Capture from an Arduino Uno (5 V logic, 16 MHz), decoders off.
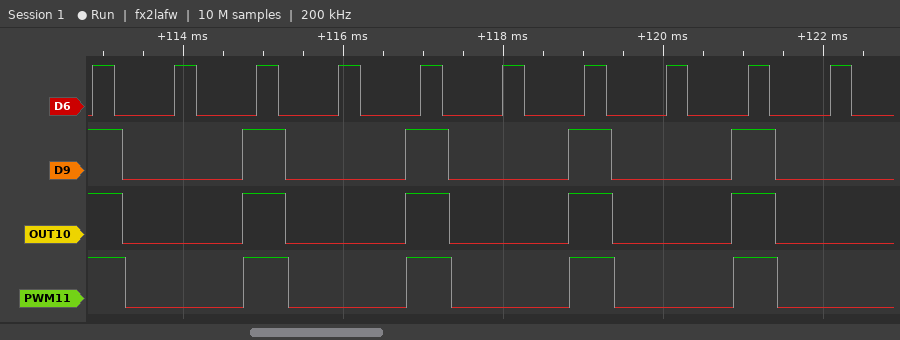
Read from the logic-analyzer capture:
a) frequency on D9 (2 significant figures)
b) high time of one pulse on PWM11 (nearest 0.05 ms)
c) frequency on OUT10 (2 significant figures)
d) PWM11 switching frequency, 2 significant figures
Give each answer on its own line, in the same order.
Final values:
490 Hz
0.55 ms
490 Hz
490 Hz
